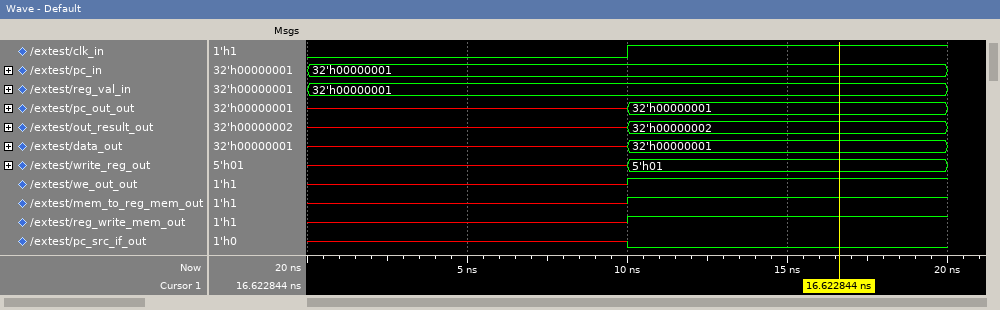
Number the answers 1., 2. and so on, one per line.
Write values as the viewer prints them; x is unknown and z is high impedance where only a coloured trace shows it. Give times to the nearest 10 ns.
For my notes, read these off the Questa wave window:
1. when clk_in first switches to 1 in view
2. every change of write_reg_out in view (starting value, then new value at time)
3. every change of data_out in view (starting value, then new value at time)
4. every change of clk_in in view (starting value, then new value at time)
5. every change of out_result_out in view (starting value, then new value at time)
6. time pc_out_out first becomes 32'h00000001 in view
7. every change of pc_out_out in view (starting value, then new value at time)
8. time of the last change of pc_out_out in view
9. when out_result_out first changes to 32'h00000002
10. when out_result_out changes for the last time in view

1. 10 ns
2. x, 5'h01 at 10 ns
3. x, 32'h00000001 at 10 ns
4. 0, 1 at 10 ns
5. x, 32'h00000002 at 10 ns
6. 10 ns
7. x, 32'h00000001 at 10 ns
8. 10 ns
9. 10 ns
10. 10 ns
